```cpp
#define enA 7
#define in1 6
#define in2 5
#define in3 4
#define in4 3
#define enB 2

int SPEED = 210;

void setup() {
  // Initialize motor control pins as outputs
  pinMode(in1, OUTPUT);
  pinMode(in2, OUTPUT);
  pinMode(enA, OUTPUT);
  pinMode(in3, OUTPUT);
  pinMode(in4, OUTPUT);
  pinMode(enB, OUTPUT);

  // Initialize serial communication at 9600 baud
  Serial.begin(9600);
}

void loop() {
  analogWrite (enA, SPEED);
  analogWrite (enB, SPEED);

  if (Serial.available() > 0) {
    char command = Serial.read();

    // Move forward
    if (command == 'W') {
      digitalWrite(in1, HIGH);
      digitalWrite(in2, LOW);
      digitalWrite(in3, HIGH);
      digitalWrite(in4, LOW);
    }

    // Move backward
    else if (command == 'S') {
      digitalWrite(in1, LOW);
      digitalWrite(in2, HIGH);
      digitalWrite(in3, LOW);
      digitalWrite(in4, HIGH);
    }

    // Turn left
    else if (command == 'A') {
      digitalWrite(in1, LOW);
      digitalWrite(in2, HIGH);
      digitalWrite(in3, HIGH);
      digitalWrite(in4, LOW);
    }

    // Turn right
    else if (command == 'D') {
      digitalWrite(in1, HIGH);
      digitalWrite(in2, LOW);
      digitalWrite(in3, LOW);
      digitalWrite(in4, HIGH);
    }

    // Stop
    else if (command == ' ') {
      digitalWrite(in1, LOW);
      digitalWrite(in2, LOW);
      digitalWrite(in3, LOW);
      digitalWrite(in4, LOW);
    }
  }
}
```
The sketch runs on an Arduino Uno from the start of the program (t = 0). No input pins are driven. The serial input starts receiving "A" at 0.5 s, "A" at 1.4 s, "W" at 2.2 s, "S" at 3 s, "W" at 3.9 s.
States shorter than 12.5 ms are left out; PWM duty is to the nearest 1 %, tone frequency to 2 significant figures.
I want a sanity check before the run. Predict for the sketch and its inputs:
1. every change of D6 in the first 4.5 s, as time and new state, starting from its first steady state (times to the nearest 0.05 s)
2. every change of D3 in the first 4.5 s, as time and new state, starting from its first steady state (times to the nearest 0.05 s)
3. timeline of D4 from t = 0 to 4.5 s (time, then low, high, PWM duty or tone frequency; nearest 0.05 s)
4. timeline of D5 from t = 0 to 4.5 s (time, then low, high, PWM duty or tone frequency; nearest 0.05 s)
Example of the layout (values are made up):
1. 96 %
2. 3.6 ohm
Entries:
1. 0 s low; 2.2 s high; 3 s low; 3.9 s high
2. 0 s low; 3 s high; 3.9 s low
3. 0 s low; 0.5 s high; 3 s low; 3.9 s high
4. 0 s low; 0.5 s high; 2.2 s low; 3 s high; 3.9 s low
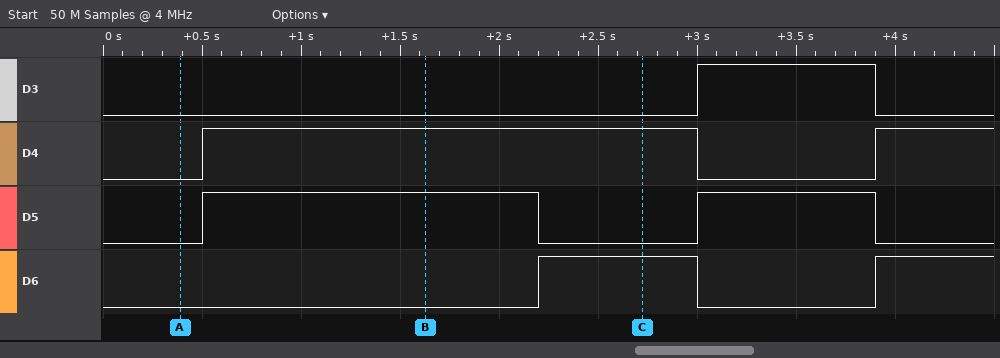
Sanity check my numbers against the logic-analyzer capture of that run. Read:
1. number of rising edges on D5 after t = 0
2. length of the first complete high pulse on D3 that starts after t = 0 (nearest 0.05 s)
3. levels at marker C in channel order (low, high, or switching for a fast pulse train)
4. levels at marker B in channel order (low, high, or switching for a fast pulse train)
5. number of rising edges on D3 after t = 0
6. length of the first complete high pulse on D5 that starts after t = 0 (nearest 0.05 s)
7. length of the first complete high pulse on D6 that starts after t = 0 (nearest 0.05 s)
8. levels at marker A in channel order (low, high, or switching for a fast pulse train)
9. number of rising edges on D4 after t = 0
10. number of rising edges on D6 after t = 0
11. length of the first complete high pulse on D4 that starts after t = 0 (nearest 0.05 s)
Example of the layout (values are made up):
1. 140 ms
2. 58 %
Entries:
1. 2
2. 0.90 s
3. D3 low, D4 high, D5 low, D6 high
4. D3 low, D4 high, D5 high, D6 low
5. 1
6. 1.70 s
7. 0.80 s
8. D3 low, D4 low, D5 low, D6 low
9. 2
10. 2
11. 2.50 s
